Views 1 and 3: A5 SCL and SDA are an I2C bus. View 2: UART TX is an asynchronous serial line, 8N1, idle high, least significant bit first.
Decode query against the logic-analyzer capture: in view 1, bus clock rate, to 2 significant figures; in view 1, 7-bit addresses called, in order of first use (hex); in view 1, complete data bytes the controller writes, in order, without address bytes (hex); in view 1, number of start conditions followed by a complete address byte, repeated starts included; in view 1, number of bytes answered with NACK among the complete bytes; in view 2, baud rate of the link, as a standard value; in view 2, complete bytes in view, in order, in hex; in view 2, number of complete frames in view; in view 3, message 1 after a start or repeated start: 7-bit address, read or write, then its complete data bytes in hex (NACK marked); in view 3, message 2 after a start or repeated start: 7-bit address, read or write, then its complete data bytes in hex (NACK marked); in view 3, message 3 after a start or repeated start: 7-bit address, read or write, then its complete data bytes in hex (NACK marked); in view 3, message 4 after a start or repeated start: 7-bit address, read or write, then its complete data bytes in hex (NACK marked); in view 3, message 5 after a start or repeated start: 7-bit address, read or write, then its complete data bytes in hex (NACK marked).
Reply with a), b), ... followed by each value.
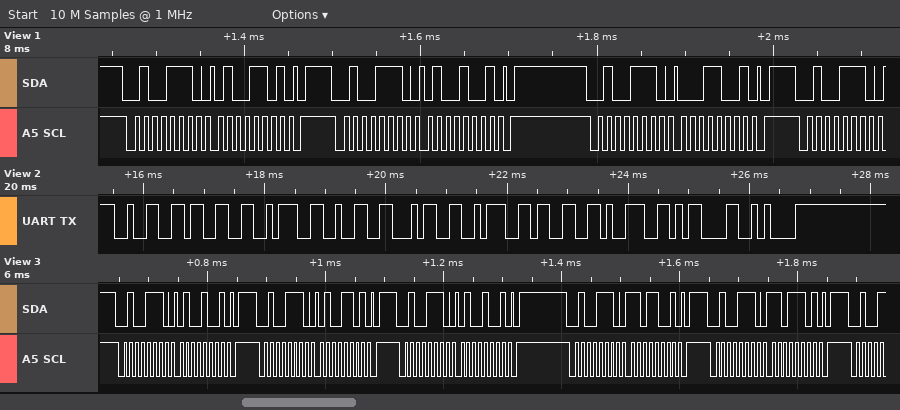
a) 100 kHz
b) 0x27
c) 4D 49 19
d) 4
e) 0
f) 9600 baud
g) 32 33 3A 32 34 3A 33 39 0D 0A
h) 10
i) 0x27 write: 49
j) 0x27 write: 4D
k) 0x27 write: 49
l) 0x27 write: D9
m) 0x27 write: DD
